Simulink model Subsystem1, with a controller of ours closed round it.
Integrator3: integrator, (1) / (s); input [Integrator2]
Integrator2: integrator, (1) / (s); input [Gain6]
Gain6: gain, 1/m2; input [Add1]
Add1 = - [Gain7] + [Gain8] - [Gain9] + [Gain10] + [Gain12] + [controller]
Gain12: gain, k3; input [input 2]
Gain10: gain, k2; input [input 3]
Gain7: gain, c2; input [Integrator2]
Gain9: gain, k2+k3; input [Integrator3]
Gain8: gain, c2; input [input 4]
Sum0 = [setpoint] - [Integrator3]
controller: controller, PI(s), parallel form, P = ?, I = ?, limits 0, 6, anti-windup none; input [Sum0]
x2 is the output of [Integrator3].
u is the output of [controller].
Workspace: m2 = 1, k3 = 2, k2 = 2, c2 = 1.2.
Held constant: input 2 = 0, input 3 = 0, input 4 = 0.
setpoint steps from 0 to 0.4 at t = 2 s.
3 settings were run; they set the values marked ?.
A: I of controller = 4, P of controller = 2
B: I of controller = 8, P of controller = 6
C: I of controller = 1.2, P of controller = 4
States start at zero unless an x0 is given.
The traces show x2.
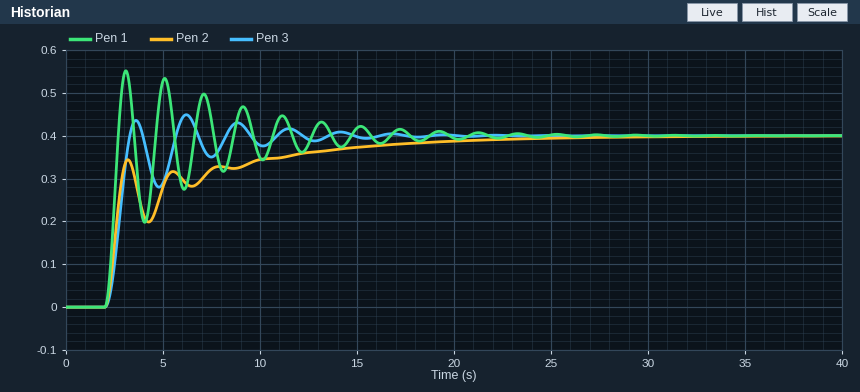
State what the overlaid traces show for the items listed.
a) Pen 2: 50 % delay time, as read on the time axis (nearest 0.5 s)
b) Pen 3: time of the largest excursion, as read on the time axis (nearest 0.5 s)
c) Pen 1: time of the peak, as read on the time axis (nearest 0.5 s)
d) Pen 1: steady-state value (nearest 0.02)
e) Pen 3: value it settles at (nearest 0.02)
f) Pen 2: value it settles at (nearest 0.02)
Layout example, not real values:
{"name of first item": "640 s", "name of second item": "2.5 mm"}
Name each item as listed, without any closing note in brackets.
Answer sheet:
{"Pen 2: 50 % delay time, as read on the time axis": "2.5 s", "Pen 3: time of the largest excursion, as read on the time axis": "6.0 s", "Pen 1: time of the peak, as read on the time axis": "3.0 s", "Pen 1: steady-state value": "0.40", "Pen 3: value it settles at": "0.40", "Pen 2: value it settles at": "0.40"}
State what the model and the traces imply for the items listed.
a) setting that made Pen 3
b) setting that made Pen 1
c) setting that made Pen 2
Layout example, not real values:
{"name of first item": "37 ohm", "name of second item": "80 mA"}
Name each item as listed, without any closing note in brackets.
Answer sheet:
{"setting that made Pen 3": "A", "setting that made Pen 1": "B", "setting that made Pen 2": "C"}
